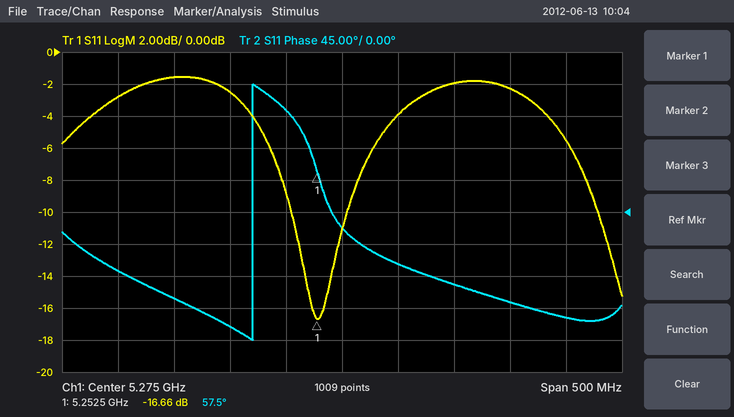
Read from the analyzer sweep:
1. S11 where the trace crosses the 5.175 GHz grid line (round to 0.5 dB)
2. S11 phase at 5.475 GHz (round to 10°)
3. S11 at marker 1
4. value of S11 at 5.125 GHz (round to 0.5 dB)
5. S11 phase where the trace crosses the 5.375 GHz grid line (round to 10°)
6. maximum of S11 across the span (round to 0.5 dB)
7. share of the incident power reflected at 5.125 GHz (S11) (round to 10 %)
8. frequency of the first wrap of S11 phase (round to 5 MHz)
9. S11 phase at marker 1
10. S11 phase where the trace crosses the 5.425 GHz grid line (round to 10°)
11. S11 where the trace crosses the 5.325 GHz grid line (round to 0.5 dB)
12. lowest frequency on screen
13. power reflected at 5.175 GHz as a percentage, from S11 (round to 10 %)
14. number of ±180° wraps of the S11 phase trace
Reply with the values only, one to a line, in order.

-2.5 dB
-150°
-16.66 dB
-1.5 dB
-100°
-1.5 dB
70 %
5.195 GHz
57.5°
-130°
-4.0 dB
5.025 GHz
60 %
1
